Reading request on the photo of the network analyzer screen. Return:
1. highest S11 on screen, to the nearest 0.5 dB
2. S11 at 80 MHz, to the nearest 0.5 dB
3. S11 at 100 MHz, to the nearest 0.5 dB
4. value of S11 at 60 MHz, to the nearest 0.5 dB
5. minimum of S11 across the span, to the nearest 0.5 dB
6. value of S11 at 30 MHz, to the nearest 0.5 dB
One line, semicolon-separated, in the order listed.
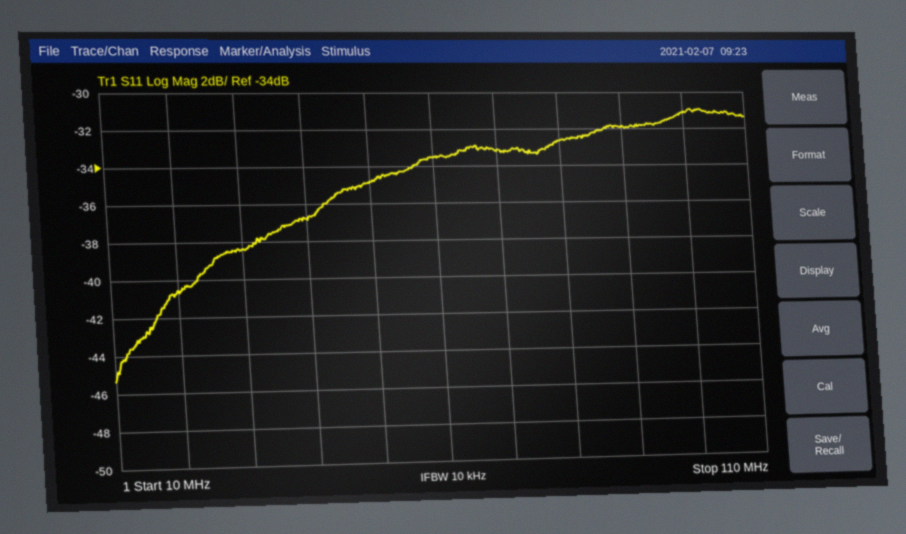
-31.0 dB; -32.5 dB; -31.0 dB; -33.5 dB; -45.5 dB; -38.5 dB
